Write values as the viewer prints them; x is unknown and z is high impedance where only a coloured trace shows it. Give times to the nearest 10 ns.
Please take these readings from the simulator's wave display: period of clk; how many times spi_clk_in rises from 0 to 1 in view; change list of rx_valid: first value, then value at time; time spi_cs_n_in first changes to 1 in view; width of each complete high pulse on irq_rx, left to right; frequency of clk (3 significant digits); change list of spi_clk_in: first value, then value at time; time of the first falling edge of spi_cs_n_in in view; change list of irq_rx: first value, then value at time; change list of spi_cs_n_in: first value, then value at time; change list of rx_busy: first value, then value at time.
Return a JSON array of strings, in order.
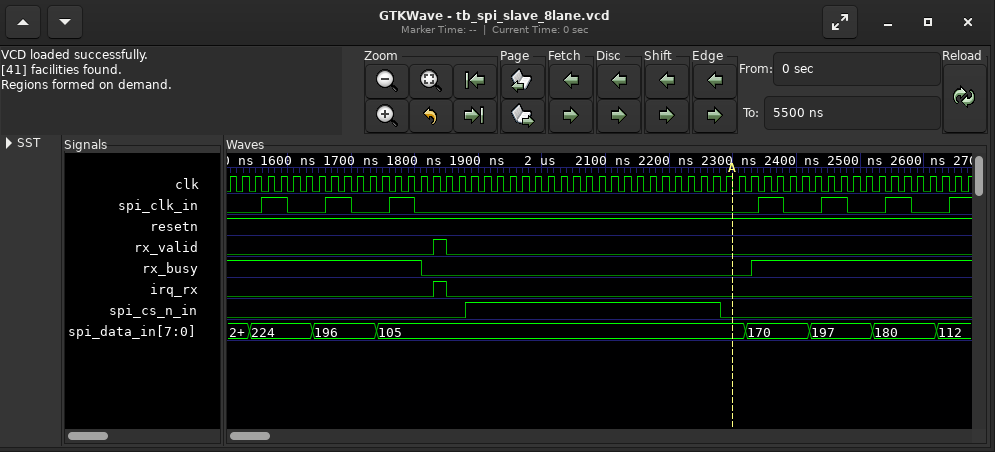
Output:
["20 ns", "7", "0, 1 at 1830 ns, 0 at 1850 ns", "1880 ns", "20 ns", "50.0 MHz", "0, 1 at 1560 ns, 0 at 1600 ns, 1 at 1660 ns, 0 at 1700 ns, 1 at 1760 ns, 0 at 1800 ns, 1 at 2340 ns, 0 at 2380 ns, 1 at 2440 ns, 0 at 2480 ns, 1 at 2540 ns, 0 at 2580 ns, 1 at 2640 ns", "2280 ns", "0, 1 at 1830 ns, 0 at 1850 ns", "0, 1 at 1880 ns, 0 at 2280 ns", "1, 0 at 1810 ns, 1 at 2330 ns"]
